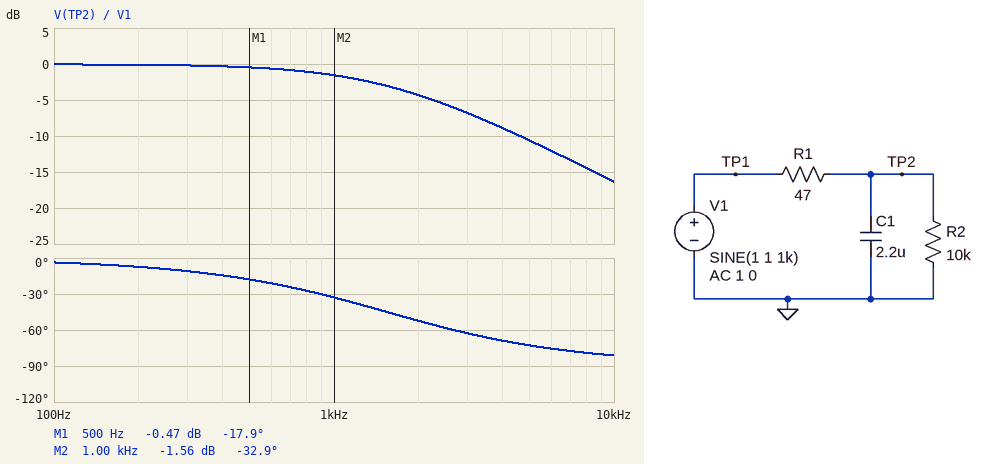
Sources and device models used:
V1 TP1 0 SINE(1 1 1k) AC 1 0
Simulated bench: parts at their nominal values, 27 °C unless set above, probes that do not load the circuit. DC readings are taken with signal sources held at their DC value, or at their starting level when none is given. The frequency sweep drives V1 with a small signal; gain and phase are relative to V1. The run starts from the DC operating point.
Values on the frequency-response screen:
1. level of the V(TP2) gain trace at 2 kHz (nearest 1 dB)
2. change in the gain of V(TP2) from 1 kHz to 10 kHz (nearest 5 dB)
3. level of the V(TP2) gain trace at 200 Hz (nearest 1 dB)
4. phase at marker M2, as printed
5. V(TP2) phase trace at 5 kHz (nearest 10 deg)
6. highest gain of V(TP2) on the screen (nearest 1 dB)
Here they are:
-4 dB
-15 dB
0 dB
-32.9 deg
-70 deg
0 dB
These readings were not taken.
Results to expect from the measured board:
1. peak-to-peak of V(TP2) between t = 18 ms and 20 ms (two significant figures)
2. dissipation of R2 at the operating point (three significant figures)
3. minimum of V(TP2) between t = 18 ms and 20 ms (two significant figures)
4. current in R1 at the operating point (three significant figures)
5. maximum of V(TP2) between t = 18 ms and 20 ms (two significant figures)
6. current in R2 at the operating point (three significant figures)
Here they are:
1.7 V
99.1 µW
160 mV
99.5 µA
1.8 V
99.5 µA
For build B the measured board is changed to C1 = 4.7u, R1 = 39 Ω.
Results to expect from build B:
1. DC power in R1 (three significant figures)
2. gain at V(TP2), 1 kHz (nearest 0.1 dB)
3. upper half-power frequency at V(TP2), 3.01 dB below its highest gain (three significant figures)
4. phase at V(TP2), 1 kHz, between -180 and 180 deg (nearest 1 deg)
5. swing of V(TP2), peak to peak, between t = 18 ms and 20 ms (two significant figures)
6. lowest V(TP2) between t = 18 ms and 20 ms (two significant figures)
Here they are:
387 nW
-3.7 dB
872 Hz
-49 deg
1.3 V
340 mV
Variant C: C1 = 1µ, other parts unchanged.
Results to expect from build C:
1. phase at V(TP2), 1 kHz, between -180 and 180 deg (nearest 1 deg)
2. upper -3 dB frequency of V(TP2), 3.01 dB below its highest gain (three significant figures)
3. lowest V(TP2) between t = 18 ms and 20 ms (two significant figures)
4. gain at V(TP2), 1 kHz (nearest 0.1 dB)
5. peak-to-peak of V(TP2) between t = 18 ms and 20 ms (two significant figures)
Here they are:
-16 deg
3.40 kHz
40 mV
-0.4 dB
1.9 V
